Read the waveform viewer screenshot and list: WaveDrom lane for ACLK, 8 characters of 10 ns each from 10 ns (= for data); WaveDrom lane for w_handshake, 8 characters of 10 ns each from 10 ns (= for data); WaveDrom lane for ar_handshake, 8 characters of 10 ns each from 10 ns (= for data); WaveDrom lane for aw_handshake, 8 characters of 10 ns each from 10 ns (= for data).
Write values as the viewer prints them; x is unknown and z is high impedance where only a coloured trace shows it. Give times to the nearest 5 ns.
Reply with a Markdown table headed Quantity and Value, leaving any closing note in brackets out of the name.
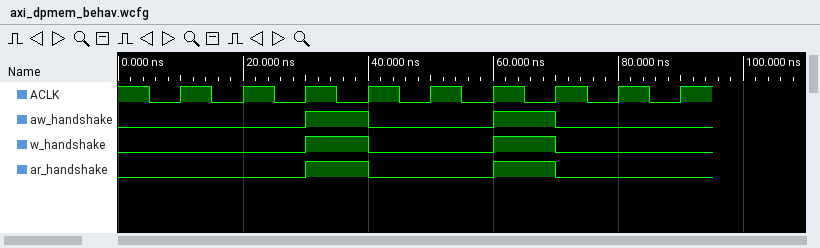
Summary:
| Quantity | Value |
|---|---|
| WaveDrom lane for ACLK, 8 characters of 10 ns each from 10 ns | {name: 'ACLK', wave: 'p.......'} |
| WaveDrom lane for w_handshake, 8 characters of 10 ns each from 10 ns | {name: 'w_handshake', wave: '0.10.10.'} |
| WaveDrom lane for ar_handshake, 8 characters of 10 ns each from 10 ns | {name: 'ar_handshake', wave: '0.10.10.'} |
| WaveDrom lane for aw_handshake, 8 characters of 10 ns each from 10 ns | {name: 'aw_handshake', wave: '0.10.10.'} |
